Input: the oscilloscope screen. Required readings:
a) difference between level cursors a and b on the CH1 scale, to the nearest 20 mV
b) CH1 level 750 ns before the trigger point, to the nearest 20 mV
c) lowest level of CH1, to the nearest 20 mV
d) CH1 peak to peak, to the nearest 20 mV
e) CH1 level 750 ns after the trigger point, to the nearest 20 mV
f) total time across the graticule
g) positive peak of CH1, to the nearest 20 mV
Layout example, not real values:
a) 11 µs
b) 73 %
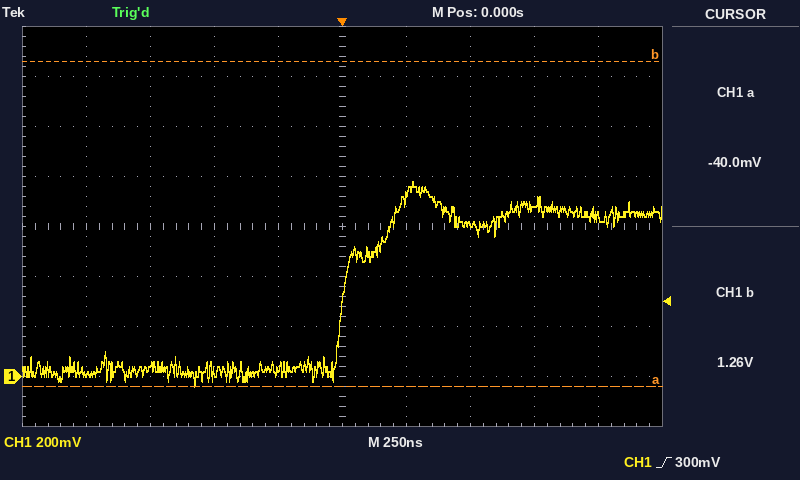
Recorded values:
a) 1.30 V
b) 40 mV
c) -40 mV
d) 820 mV
e) 680 mV
f) 2.5 µs
g) 780 mV
